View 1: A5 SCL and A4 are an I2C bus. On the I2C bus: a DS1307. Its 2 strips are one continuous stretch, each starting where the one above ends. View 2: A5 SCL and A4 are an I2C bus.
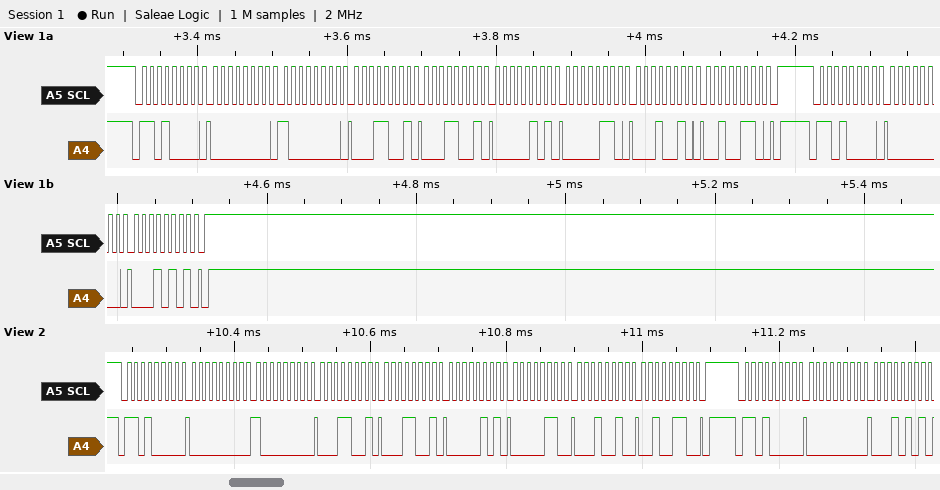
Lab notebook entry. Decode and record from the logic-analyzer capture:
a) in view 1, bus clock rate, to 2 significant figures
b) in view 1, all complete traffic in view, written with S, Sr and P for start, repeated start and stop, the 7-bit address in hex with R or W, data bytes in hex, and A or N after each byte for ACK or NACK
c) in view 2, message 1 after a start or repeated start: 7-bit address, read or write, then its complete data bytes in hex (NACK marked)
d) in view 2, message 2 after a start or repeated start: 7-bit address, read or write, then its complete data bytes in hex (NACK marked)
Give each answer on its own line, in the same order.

100 kHz
S 68W A 00 A 80 A 19 A 19 A 05 A 06 A 12 A 26 A P S 68W A 00 A 15 A P
0x68 write: 00 80 19 19 05 06 12 26
0x68 write: 00 15
